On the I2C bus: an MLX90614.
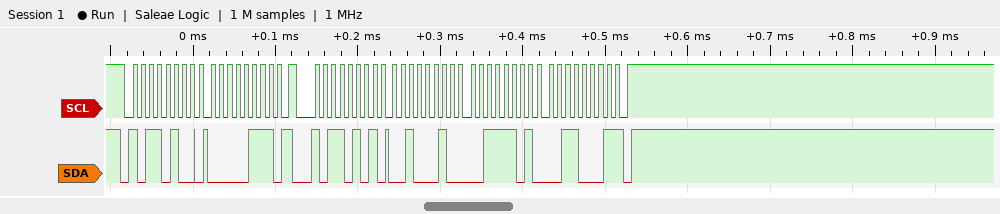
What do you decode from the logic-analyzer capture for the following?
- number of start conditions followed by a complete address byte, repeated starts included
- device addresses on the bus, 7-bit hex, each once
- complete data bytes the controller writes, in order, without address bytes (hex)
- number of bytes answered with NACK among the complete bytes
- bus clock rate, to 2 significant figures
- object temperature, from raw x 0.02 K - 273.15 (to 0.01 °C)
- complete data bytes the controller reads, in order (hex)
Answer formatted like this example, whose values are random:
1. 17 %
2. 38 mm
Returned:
1. 2
2. 0x5A
3. 07
4. 1
5. 100 kHz
6. 39.85 °C
7. 22 3D 31
